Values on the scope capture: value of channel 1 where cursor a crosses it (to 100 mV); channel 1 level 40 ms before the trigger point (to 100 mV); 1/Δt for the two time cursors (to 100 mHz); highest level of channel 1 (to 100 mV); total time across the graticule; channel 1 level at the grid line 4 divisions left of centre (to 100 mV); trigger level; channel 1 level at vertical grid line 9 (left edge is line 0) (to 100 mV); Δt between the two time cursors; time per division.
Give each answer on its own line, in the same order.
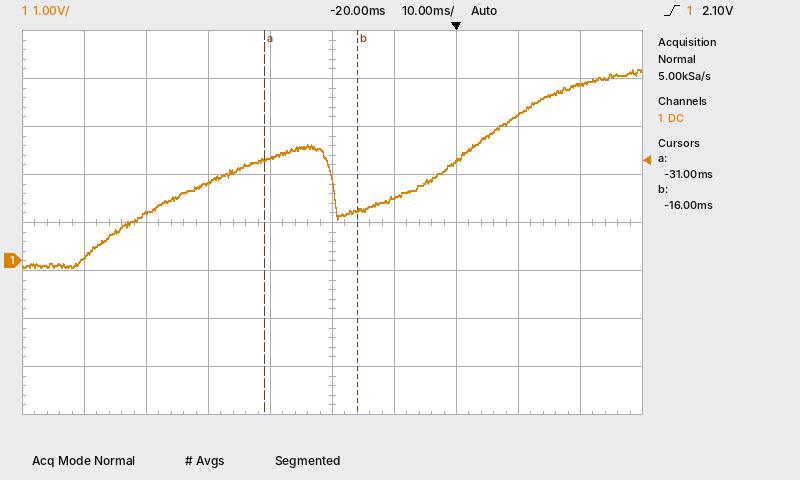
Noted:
2.1 V
1.6 V
66.7 Hz
4.0 V
100 ms
100 mV
2.10 V
3.7 V
15 ms
10 ms
